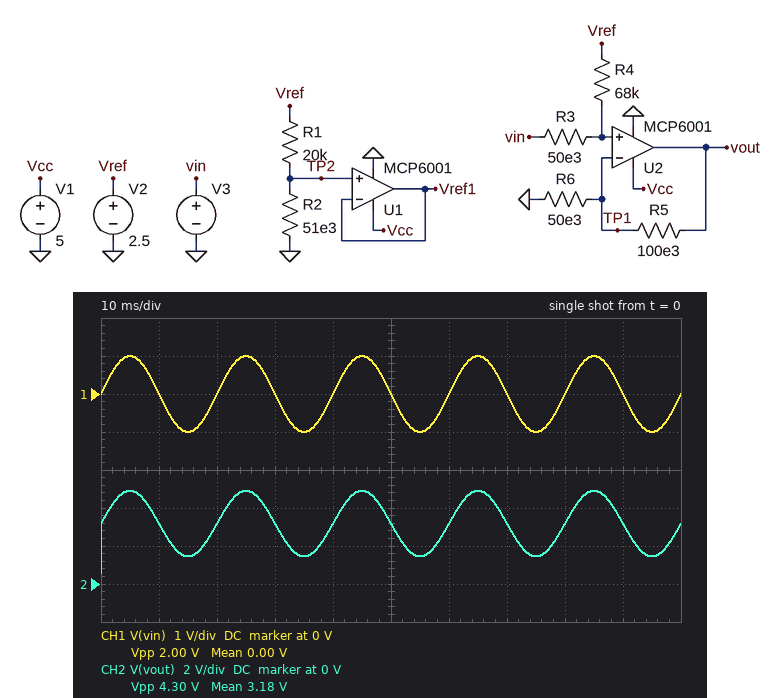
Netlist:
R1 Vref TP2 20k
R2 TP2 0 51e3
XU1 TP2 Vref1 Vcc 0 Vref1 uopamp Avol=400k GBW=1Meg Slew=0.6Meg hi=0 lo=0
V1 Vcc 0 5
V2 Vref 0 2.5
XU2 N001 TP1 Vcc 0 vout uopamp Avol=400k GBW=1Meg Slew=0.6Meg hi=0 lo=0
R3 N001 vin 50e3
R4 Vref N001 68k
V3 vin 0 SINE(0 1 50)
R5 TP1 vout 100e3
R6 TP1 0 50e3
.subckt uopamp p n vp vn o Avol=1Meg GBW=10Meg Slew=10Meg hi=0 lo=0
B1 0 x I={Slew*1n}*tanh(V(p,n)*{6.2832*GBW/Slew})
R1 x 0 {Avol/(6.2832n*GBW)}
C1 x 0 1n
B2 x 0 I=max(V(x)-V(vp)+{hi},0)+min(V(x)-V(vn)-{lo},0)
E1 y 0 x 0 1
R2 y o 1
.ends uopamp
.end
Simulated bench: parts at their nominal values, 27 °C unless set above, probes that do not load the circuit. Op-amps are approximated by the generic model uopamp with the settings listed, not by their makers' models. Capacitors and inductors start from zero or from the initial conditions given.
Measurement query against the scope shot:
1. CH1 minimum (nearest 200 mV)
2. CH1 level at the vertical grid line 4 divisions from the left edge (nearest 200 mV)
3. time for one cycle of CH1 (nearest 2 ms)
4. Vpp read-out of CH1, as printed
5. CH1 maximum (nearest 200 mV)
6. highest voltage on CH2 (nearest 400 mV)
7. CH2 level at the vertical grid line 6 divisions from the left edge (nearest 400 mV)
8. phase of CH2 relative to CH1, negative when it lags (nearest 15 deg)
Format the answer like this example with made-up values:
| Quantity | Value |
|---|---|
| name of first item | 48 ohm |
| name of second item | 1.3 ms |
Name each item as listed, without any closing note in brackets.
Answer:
| Quantity | Value |
|---|---|
| CH1 minimum | -1.0 V |
| CH1 level at the vertical grid line 4 divisions from the left edge | 0 V |
| time for one cycle of CH1 | 20 ms |
| Vpp read-out of CH1, as printed | 2.00 V |
| CH1 maximum | 1.0 V |
| highest voltage on CH2 | 4.8 V |
| CH2 level at the vertical grid line 6 divisions from the left edge | 3.2 V |
| phase of CH2 relative to CH1, negative when it lags | 0 deg |
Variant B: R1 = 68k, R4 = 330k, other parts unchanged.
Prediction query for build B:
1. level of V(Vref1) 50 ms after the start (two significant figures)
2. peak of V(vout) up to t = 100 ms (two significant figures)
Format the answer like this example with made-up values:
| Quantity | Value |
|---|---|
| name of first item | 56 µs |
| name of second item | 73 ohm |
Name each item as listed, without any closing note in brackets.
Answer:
| Quantity | Value |
|---|---|
| level of V(Vref1) 50 ms after the start | 1.1 V |
| peak of V(vout) up to t = 100 ms | 3.6 V |
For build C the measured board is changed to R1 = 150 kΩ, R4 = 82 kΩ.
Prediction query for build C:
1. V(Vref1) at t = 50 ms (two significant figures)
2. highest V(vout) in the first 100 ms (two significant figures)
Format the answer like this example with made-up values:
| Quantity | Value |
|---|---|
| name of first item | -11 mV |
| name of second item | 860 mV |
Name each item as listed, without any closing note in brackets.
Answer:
| Quantity | Value |
|---|---|
| V(Vref1) at t = 50 ms | 630 mV |
| highest V(vout) in the first 100 ms | 4.7 V |
